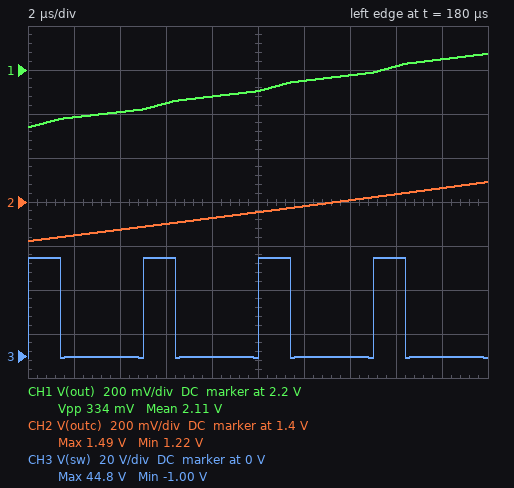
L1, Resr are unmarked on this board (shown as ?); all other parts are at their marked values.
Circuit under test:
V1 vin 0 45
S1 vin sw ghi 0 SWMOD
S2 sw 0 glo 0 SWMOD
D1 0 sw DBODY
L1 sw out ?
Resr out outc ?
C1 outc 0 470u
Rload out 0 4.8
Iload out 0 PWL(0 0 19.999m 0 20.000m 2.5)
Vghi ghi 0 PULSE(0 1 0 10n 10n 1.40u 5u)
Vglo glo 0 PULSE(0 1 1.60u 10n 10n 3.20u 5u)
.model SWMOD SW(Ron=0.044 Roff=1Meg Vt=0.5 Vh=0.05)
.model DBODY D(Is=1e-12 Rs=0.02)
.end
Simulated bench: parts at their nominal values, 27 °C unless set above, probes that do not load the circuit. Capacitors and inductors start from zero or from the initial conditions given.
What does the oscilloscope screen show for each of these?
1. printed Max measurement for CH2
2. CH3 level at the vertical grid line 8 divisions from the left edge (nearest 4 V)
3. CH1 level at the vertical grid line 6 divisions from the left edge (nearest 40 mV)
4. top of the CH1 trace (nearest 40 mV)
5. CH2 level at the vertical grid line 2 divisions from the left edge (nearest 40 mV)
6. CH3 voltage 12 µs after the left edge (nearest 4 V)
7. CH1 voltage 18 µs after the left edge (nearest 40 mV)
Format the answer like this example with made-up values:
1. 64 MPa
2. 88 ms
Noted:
1. 1.49 V
2. 44 V
3. 2.16 V
4. 2.28 V
5. 1.28 V
6. 0 V
7. 2.24 V
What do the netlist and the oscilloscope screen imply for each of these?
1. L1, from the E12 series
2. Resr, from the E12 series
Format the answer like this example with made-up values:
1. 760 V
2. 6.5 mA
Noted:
1. 330 µH
2. 0.12 Ω
